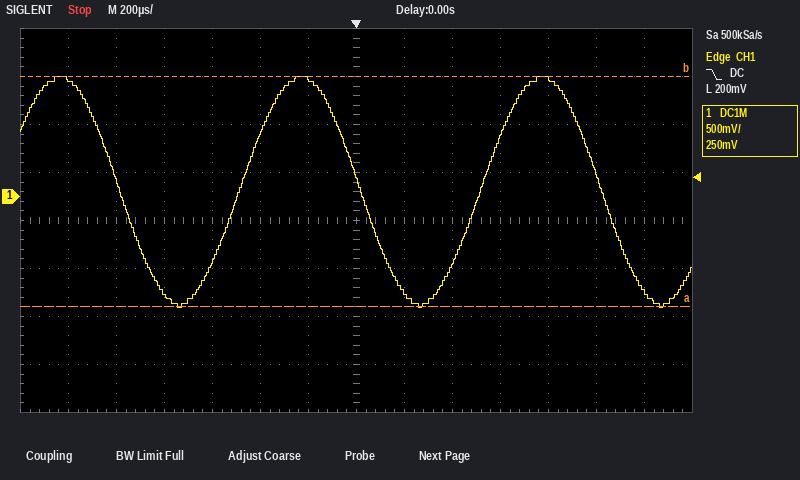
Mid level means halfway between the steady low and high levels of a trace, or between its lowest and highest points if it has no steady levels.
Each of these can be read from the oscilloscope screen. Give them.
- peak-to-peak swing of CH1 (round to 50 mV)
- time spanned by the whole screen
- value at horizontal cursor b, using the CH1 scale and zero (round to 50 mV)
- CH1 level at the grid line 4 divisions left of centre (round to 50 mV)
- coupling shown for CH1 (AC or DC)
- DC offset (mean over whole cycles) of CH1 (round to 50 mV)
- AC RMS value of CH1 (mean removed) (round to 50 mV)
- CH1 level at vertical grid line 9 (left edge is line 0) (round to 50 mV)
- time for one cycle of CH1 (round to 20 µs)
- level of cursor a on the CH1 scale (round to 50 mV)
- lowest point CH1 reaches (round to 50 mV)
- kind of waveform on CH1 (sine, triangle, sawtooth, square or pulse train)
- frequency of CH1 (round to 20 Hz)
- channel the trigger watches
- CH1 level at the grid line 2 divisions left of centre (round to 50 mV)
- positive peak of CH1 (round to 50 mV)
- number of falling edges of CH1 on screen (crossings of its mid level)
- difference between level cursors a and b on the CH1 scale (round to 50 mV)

2.40 V
2.8 ms
1.25 V
-1.00 V
DC
50 mV
850 mV
-700 mV
1.00 ms
-1.15 V
-1.15 V
sine
1.00 kHz
CH1
650 mV
1.25 V
3
2.40 V
